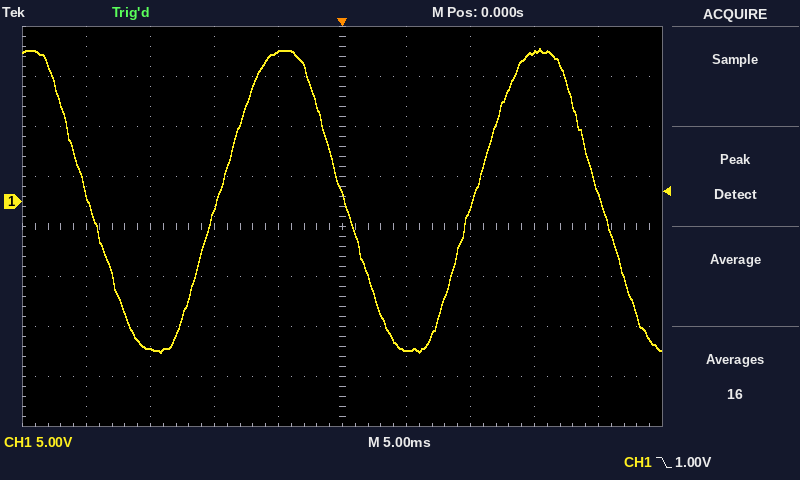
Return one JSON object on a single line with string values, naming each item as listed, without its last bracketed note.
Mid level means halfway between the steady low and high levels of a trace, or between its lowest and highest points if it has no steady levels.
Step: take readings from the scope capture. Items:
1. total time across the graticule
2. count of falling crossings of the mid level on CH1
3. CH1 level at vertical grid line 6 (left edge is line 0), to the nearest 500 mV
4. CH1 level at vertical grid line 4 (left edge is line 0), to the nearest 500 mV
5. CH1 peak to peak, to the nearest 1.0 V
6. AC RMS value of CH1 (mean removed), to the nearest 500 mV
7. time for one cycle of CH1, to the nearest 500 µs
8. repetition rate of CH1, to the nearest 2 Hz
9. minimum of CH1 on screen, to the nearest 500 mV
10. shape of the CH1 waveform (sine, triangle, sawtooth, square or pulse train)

{"total time across the graticule": "50 ms", "count of falling crossings of the mid level on CH1": "3", "CH1 level at vertical grid line 6 (left edge is line 0), to the nearest 500 mV": "-15.0 V", "CH1 level at vertical grid line 4 (left edge is line 0), to the nearest 500 mV": "15.0 V", "CH1 peak to peak, to the nearest 1.0 V": "30.0 V", "AC RMS value of CH1 (mean removed), to the nearest 500 mV": "10.5 V", "time for one cycle of CH1, to the nearest 500 µs": "20.0 ms", "repetition rate of CH1, to the nearest 2 Hz": "50 Hz", "minimum of CH1 on screen, to the nearest 500 mV": "-15.0 V", "shape of the CH1 waveform": "sine"}
